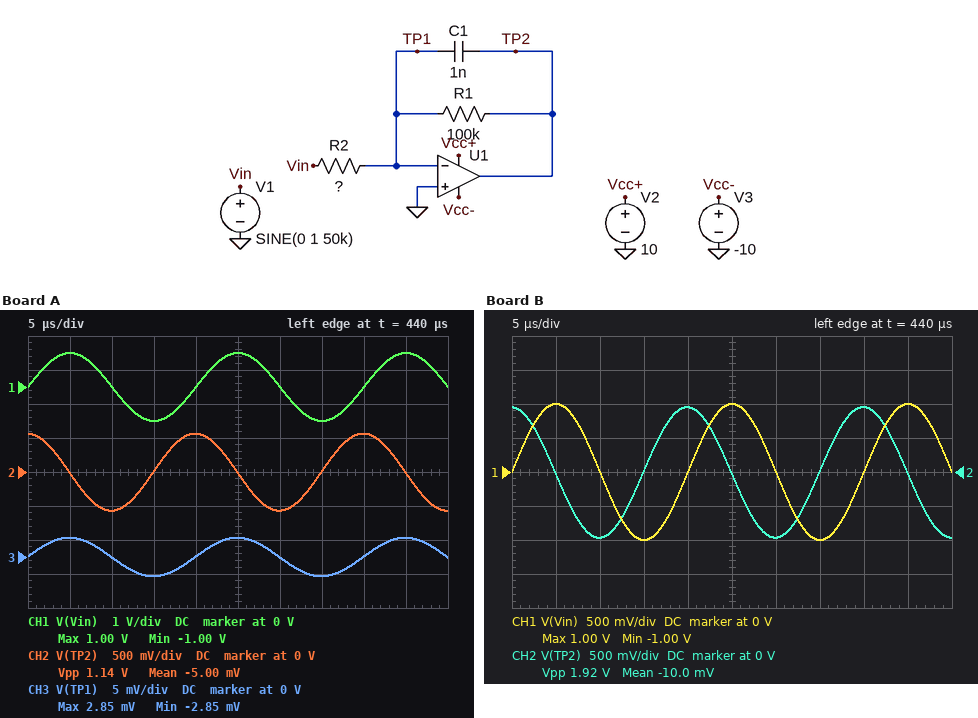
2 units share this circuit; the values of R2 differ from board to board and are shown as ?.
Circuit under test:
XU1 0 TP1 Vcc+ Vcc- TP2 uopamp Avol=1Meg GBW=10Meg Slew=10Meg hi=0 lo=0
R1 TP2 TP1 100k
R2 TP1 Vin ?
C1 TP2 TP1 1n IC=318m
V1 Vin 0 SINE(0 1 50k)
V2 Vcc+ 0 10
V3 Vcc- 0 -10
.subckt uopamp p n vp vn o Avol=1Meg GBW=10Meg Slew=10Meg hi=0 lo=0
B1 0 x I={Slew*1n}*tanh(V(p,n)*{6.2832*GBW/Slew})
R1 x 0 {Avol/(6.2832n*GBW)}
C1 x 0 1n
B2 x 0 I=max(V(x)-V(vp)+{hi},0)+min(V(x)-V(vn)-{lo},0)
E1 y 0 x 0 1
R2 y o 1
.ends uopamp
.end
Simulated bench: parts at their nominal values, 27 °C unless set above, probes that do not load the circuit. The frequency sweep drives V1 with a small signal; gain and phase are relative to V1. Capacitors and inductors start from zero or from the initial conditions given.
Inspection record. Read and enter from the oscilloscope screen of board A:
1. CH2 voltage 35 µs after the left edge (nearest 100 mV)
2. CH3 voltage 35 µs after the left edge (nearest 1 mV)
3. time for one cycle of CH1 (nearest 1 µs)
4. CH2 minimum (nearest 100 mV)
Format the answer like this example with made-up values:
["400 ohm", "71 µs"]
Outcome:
["0 V", "-3 mV", "20 µs", "-600 mV"]
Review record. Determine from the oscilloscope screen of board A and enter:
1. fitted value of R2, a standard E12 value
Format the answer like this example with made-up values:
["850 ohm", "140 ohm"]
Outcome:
["5.6 kΩ"]
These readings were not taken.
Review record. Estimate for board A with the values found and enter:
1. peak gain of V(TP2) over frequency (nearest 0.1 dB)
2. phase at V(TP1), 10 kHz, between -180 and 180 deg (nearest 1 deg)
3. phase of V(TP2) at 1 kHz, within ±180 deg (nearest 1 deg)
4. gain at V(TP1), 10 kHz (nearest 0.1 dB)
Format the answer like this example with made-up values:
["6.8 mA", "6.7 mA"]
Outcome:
["25.0 dB", "9 deg", "148 deg", "-51.1 dB"]
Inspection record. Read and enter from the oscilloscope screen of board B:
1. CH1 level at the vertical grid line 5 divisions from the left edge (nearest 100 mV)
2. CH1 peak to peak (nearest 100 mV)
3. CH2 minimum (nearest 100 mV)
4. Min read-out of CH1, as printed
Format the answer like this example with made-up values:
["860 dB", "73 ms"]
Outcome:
["1.0 V", "2.0 V", "-1.0 V", "-1.00 V"]
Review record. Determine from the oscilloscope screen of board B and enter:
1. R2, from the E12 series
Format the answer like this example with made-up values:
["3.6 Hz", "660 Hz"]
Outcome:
["3.3 kΩ"]
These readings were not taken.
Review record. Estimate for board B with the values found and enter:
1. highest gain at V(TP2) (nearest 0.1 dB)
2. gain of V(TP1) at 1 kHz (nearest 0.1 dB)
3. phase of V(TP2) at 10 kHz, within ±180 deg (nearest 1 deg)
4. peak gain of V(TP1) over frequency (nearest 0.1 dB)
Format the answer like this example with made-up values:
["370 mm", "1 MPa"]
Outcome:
["29.6 dB", "-51.8 dB", "99 deg", "-46.4 dB"]
